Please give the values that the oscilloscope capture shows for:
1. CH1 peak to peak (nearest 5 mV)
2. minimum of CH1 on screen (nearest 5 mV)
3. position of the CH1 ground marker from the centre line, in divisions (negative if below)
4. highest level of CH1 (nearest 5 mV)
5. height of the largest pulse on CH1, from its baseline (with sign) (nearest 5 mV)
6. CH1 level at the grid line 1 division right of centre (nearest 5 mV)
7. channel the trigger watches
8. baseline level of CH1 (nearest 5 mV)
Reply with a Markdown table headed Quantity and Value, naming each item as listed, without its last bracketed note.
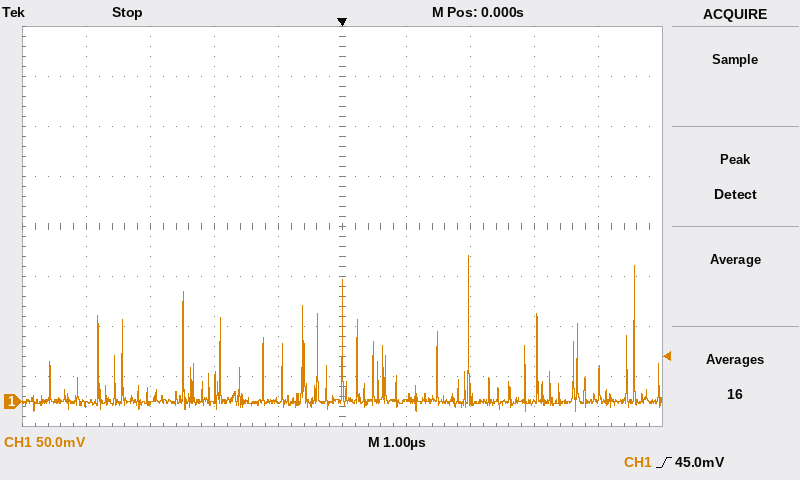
| Quantity | Value |
|---|---|
| CH1 peak to peak | 155 mV |
| minimum of CH1 on screen | -10 mV |
| position of the CH1 ground marker from the centre line, in divisions | -3.5 div |
| highest level of CH1 | 145 mV |
| height of the largest pulse on CH1, from its baseline (with sign) | +145 mV |
| CH1 level at the grid line 1 division right of centre | 5 mV |
| channel the trigger watches | CH1 |
| baseline level of CH1 | 0 mV |
